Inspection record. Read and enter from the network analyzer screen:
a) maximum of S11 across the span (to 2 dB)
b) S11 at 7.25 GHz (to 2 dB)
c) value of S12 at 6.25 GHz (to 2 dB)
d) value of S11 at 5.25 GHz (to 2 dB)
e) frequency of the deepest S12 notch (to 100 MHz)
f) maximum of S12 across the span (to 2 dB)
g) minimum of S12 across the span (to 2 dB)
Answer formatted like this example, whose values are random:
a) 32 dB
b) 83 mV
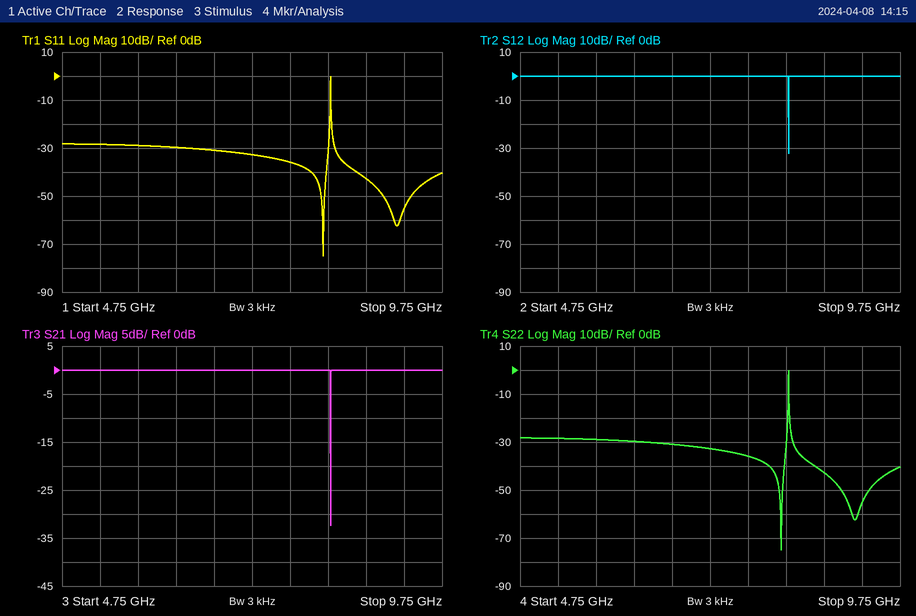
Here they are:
a) 0 dB
b) -32 dB
c) 0 dB
d) -28 dB
e) 8.3 GHz
f) 0 dB
g) -32 dB
